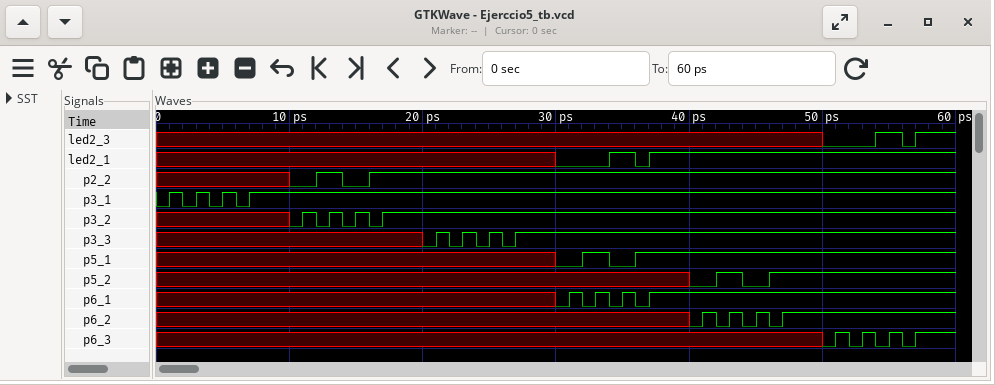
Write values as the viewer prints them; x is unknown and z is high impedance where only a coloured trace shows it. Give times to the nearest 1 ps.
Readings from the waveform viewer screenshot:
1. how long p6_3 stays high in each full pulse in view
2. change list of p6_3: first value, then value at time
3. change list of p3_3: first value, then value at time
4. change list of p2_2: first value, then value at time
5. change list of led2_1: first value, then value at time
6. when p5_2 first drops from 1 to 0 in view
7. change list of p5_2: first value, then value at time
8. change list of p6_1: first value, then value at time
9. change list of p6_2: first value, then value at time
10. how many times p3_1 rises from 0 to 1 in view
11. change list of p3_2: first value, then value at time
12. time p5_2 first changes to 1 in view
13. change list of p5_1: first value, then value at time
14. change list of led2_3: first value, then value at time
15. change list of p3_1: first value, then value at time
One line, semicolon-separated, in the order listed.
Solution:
1 ps, 1 ps, 1 ps; x, 0 at 50 ps, 1 at 51 ps, 0 at 52 ps, 1 at 53 ps, 0 at 54 ps, 1 at 55 ps, 0 at 56 ps, 1 at 57 ps; x, 0 at 20 ps, 1 at 21 ps, 0 at 22 ps, 1 at 23 ps, 0 at 24 ps, 1 at 25 ps, 0 at 26 ps, 1 at 27 ps; x, 0 at 10 ps, 1 at 12 ps, 0 at 14 ps, 1 at 16 ps; x, 0 at 30 ps, 1 at 34 ps, 0 at 36 ps, 1 at 37 ps; 44 ps; x, 0 at 40 ps, 1 at 42 ps, 0 at 44 ps, 1 at 46 ps; x, 0 at 30 ps, 1 at 31 ps, 0 at 32 ps, 1 at 33 ps, 0 at 34 ps, 1 at 35 ps, 0 at 36 ps, 1 at 37 ps; x, 0 at 40 ps, 1 at 41 ps, 0 at 42 ps, 1 at 43 ps, 0 at 44 ps, 1 at 45 ps, 0 at 46 ps, 1 at 47 ps; 4; x, 0 at 10 ps, 1 at 11 ps, 0 at 12 ps, 1 at 13 ps, 0 at 14 ps, 1 at 15 ps, 0 at 16 ps, 1 at 17 ps; 42 ps; x, 0 at 30 ps, 1 at 32 ps, 0 at 34 ps, 1 at 36 ps; x, 0 at 50 ps, 1 at 54 ps, 0 at 56 ps, 1 at 57 ps; 0, 1 at 1 ps, 0 at 2 ps, 1 at 3 ps, 0 at 4 ps, 1 at 5 ps, 0 at 6 ps, 1 at 7 ps
